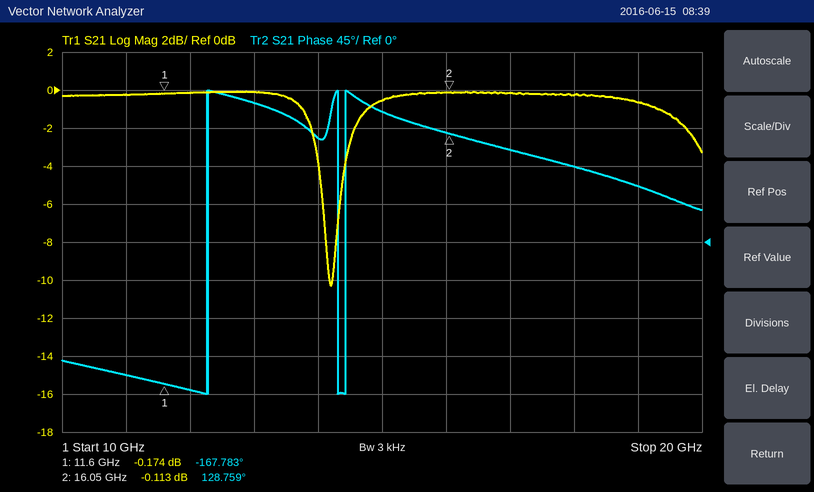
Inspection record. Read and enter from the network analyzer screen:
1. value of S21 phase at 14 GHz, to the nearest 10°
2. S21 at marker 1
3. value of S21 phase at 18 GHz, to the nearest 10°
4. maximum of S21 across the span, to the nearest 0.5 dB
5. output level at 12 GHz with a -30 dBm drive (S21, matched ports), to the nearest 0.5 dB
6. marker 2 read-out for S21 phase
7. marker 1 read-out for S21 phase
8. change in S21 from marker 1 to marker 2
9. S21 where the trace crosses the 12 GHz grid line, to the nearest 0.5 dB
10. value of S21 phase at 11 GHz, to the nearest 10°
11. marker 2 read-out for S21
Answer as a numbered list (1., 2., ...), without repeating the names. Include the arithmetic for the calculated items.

1. 120°
2. -0.174 dB
3. 90°
4. 0.0 dB
5. -30 dBm + (0.0 dB) = -30.0 dBm
6. 128.759°
7. -167.783°
8. -0.113 − (-0.174) = 0.061 dB
9. 0.0 dB
10. -160°
11. -0.113 dB
